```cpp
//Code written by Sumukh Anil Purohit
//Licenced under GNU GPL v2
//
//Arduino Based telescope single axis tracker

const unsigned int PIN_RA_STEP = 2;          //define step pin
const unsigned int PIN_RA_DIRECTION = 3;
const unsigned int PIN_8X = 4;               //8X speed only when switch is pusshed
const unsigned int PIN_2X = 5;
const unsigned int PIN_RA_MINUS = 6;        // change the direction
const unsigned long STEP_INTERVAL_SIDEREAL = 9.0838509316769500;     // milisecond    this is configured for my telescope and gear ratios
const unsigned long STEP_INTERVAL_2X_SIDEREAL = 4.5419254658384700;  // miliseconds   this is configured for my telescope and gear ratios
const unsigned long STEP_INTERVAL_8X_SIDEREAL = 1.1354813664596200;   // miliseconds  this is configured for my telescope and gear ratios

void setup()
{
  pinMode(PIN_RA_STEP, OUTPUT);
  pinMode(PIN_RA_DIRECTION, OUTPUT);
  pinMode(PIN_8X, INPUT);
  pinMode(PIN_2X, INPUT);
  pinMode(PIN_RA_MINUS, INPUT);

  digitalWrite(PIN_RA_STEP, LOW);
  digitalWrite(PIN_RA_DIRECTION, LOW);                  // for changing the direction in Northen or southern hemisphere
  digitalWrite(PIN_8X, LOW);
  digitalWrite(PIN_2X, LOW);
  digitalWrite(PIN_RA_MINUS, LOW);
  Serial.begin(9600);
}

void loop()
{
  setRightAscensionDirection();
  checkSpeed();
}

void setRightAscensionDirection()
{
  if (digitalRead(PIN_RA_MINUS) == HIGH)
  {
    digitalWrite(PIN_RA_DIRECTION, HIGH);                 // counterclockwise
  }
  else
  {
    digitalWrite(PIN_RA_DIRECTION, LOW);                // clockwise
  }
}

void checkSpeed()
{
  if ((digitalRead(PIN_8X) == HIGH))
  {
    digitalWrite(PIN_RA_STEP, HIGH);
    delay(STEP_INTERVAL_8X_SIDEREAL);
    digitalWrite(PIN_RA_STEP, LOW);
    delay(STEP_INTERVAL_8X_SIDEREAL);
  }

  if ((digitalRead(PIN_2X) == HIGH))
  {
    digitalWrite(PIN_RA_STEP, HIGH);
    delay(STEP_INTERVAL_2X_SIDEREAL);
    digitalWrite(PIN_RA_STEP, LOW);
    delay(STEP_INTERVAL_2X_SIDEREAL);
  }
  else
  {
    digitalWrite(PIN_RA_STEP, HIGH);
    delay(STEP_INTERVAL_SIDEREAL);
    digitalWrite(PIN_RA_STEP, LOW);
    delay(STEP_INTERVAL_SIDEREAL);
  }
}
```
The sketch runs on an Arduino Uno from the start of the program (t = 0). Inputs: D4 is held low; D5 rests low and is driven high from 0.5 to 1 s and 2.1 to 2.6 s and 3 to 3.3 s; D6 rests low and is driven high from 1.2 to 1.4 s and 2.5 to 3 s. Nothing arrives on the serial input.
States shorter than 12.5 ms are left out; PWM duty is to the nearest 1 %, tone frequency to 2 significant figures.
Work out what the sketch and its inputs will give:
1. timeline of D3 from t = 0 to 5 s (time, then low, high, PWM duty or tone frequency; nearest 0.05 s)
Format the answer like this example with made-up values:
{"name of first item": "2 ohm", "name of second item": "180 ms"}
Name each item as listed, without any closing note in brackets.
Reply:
{"timeline of D3 from t = 0 to 5 s": "0 s low; 1.2 s high; 1.4 s low; 2.5 s high; 3 s low"}
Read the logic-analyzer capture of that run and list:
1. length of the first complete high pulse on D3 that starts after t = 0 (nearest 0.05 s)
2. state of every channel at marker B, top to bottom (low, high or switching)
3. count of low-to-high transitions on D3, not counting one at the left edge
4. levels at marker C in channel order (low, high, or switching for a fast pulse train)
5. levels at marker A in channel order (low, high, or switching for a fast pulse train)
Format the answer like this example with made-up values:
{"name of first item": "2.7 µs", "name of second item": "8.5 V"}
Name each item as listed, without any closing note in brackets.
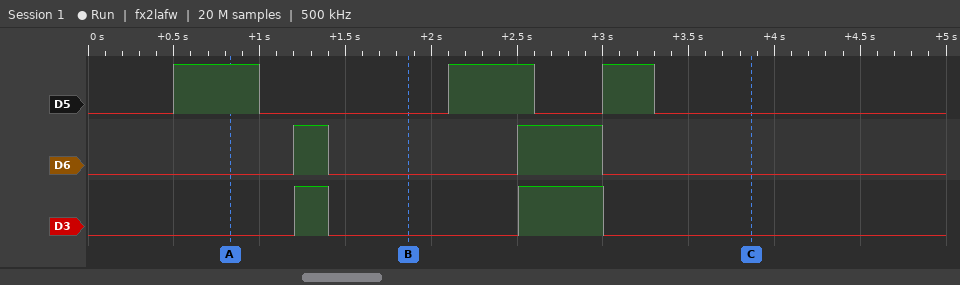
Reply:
{"length of the first complete high pulse on D3 that starts after t = 0": "0.20 s", "state of every channel at marker B, top to bottom": "D5 low, D6 low, D3 low", "count of low-to-high transitions on D3, not counting one at the left edge": "2", "levels at marker C in channel order": "D5 low, D6 low, D3 low", "levels at marker A in channel order": "D5 high, D6 low, D3 low"}
